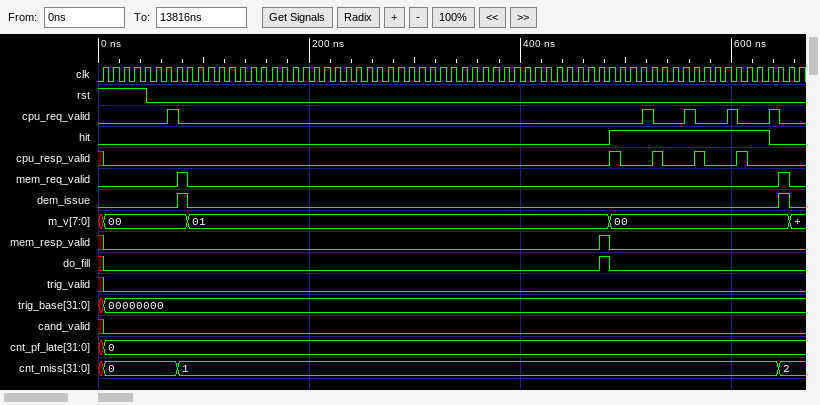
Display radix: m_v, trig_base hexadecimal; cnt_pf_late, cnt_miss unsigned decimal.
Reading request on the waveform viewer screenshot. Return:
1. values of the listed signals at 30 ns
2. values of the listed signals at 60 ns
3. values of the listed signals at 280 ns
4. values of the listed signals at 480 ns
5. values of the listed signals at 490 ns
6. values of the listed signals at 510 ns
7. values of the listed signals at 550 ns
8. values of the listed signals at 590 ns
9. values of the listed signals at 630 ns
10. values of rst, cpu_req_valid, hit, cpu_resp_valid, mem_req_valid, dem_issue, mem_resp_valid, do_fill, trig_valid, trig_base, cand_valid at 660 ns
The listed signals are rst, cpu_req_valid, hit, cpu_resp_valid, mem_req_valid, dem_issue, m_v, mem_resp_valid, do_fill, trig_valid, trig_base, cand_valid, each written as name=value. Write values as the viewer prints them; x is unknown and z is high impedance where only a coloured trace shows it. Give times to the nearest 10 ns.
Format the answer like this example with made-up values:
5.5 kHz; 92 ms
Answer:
rst=1, cpu_req_valid=0, hit=0, cpu_resp_valid=0, mem_req_valid=0, dem_issue=0, m_v=00, mem_resp_valid=0, do_fill=0, trig_valid=0, trig_base=00000000, cand_valid=0; rst=0, cpu_req_valid=0, hit=0, cpu_resp_valid=0, mem_req_valid=0, dem_issue=0, m_v=00, mem_resp_valid=0, do_fill=0, trig_valid=0, trig_base=00000000, cand_valid=0; rst=0, cpu_req_valid=0, hit=0, cpu_resp_valid=0, mem_req_valid=0, dem_issue=0, m_v=01, mem_resp_valid=0, do_fill=0, trig_valid=0, trig_base=00000000, cand_valid=0; rst=0, cpu_req_valid=0, hit=0, cpu_resp_valid=0, mem_req_valid=0, dem_issue=0, m_v=01, mem_resp_valid=1, do_fill=1, trig_valid=0, trig_base=00000000, cand_valid=0; rst=0, cpu_req_valid=0, hit=1, cpu_resp_valid=1, mem_req_valid=0, dem_issue=0, m_v=00, mem_resp_valid=0, do_fill=0, trig_valid=0, trig_base=00000000, cand_valid=0; rst=0, cpu_req_valid=0, hit=1, cpu_resp_valid=0, mem_req_valid=0, dem_issue=0, m_v=00, mem_resp_valid=0, do_fill=0, trig_valid=0, trig_base=00000000, cand_valid=0; rst=0, cpu_req_valid=0, hit=1, cpu_resp_valid=0, mem_req_valid=0, dem_issue=0, m_v=00, mem_resp_valid=0, do_fill=0, trig_valid=0, trig_base=00000000, cand_valid=0; rst=0, cpu_req_valid=0, hit=1, cpu_resp_valid=0, mem_req_valid=0, dem_issue=0, m_v=00, mem_resp_valid=0, do_fill=0, trig_valid=0, trig_base=00000000, cand_valid=0; rst=0, cpu_req_valid=0, hit=1, cpu_resp_valid=0, mem_req_valid=0, dem_issue=0, m_v=00, mem_resp_valid=0, do_fill=0, trig_valid=0, trig_base=00000000, cand_valid=0; rst=0, cpu_req_valid=0, hit=0, cpu_resp_valid=0, mem_req_valid=0, dem_issue=0, mem_resp_valid=0, do_fill=0, trig_valid=0, trig_base=00000000, cand_valid=0
